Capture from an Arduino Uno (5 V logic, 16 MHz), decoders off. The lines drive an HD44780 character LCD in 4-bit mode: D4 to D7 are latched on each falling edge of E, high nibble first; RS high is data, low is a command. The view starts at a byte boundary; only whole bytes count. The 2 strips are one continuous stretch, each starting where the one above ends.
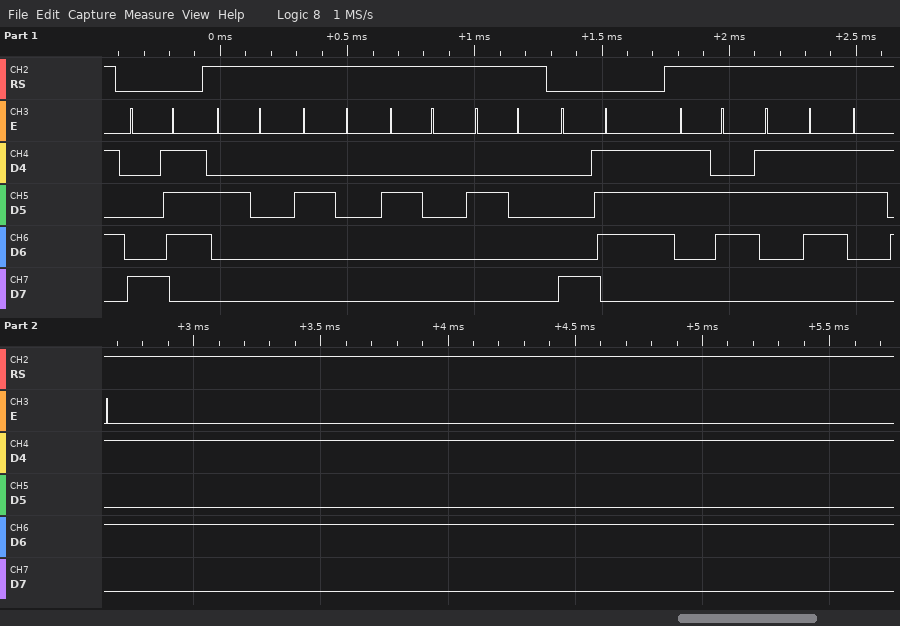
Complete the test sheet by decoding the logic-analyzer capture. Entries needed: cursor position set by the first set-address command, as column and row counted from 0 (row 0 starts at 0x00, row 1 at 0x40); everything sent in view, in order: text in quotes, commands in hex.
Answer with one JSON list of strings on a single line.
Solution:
["column 7, row 0", "0x87 \"    \" 0x87 \"675\""]
